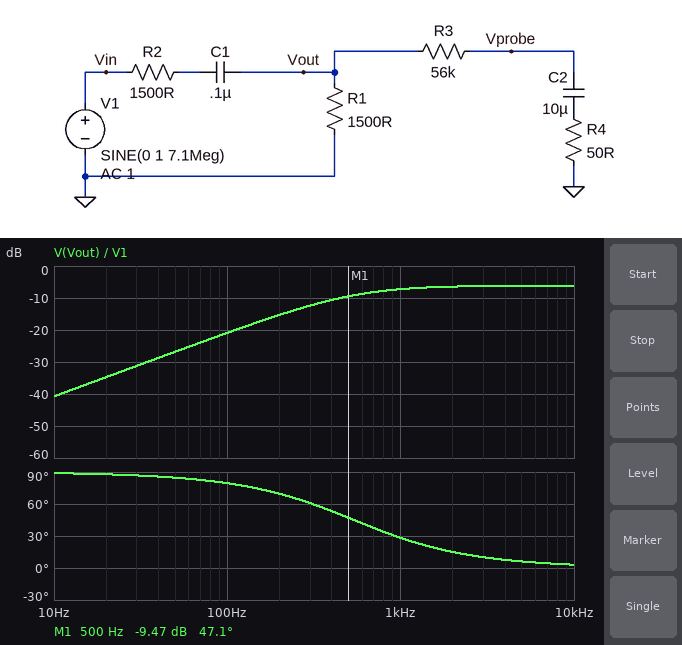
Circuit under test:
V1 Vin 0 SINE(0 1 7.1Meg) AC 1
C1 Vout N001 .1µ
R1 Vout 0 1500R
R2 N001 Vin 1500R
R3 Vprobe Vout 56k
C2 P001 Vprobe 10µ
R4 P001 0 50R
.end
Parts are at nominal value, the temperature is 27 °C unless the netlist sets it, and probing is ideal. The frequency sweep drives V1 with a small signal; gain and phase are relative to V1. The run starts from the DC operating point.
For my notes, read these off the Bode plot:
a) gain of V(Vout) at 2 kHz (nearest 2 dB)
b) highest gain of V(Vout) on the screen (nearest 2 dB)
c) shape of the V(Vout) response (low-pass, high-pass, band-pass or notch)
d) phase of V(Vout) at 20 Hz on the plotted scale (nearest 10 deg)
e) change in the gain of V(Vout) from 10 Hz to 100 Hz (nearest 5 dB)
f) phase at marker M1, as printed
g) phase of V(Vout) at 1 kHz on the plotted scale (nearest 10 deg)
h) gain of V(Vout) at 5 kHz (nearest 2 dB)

-6 dB
-6 dB
high-pass
90 deg
20 dB
47.1 deg
30 deg
-6 dB
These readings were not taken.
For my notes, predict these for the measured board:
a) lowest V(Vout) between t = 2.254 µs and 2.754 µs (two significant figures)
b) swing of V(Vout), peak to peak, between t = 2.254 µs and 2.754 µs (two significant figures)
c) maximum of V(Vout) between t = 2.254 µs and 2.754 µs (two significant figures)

-490 mV
990 mV
490 mV
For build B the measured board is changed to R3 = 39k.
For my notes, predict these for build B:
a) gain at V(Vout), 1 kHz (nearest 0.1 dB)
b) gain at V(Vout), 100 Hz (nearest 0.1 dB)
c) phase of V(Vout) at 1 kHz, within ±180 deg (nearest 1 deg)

-7.3 dB
-21.0 dB
28 deg
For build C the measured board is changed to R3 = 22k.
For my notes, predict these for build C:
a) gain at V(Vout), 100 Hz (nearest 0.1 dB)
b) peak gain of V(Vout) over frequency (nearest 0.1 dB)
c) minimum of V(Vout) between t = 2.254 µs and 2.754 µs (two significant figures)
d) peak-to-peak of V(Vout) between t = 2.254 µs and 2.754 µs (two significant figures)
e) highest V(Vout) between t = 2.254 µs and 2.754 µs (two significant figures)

-21.2 dB
-6.3 dB
-480 mV
970 mV
480 mV
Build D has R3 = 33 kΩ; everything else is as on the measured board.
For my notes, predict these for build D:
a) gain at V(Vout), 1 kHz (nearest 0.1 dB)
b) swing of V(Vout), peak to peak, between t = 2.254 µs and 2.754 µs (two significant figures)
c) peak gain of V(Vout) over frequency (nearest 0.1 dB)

-7.3 dB
980 mV
-6.2 dB
